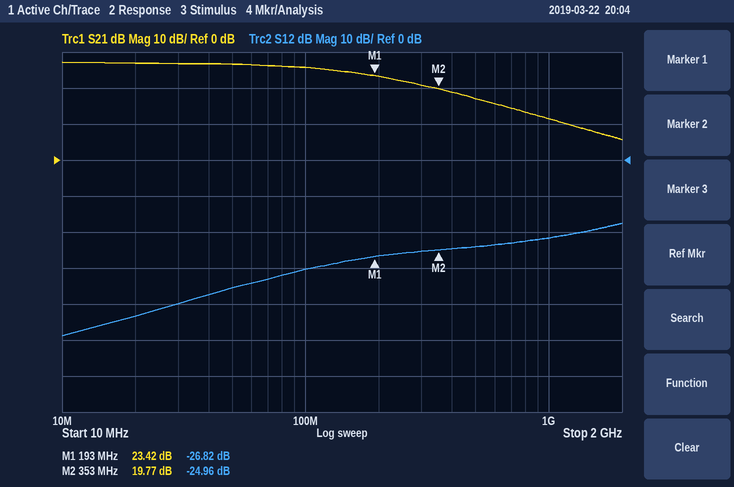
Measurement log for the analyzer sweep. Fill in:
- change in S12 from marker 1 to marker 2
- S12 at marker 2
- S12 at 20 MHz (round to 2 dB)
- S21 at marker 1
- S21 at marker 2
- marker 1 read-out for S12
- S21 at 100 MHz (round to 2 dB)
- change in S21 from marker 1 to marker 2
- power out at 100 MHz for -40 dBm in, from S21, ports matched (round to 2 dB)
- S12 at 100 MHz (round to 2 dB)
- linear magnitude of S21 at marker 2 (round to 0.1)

1.86 dB
-24.96 dB
-44 dB
23.42 dB
19.77 dB
-26.82 dB
26 dB
-3.65 dB
-14 dBm
-30 dB
9.7
